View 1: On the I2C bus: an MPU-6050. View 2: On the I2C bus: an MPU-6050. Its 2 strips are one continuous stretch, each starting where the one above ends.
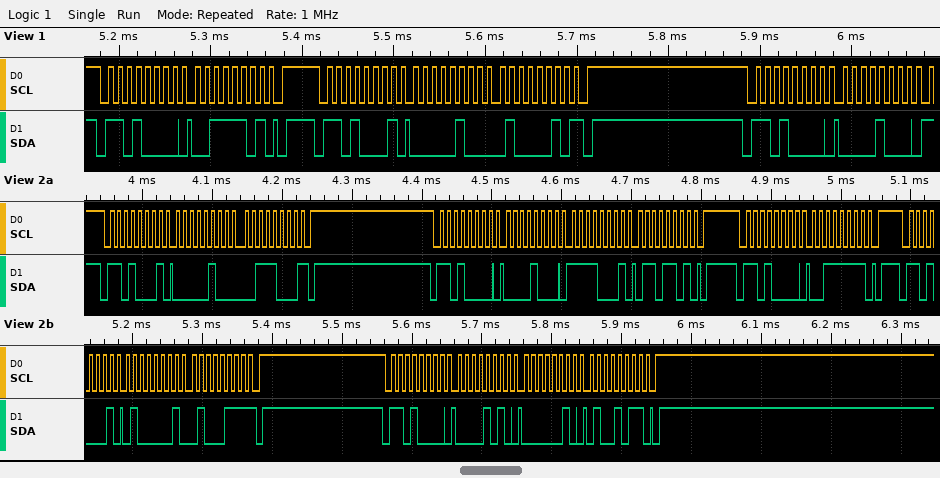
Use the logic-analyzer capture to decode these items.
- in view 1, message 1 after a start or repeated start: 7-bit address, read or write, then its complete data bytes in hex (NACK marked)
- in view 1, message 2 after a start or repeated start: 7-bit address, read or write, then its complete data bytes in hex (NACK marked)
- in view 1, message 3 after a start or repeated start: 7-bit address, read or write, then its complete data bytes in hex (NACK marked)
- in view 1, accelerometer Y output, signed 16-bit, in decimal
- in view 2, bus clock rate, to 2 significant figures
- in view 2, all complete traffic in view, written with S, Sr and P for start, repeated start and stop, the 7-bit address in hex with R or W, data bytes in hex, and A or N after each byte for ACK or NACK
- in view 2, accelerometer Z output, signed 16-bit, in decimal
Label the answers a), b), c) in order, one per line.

a) 0x68 write: 3D
b) 0x68 read: 04 42 NACK
c) 0x68 write: 08
d) 1090
e) 100 kHz
f) S 68R A 04 A 38 N P S 68W A 08 A F1 A 6D A P S 68W A 3F A P S 68R A 41 A 47 N P S 68W A 0A A 02 A 4B A P
g) 16711
